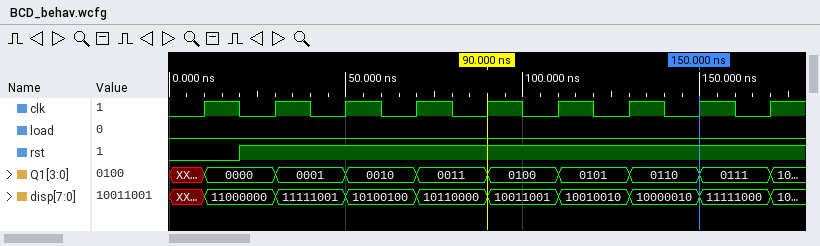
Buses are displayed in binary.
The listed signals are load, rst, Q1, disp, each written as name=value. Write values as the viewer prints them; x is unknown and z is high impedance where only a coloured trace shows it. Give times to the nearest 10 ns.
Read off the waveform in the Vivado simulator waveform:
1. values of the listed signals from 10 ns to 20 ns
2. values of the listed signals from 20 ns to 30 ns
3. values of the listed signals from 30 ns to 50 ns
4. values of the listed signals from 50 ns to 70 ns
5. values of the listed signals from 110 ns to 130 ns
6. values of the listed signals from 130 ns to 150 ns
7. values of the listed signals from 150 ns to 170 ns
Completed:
load=0, rst=0, Q1=0000, disp=11000000
load=0, rst=1, Q1=0000, disp=11000000
load=0, rst=1, Q1=0001, disp=11111001
load=0, rst=1, Q1=0010, disp=10100100
load=0, rst=1, Q1=0101, disp=10010010
load=0, rst=1, Q1=0110, disp=10000010
load=0, rst=1, Q1=0111, disp=11111000
